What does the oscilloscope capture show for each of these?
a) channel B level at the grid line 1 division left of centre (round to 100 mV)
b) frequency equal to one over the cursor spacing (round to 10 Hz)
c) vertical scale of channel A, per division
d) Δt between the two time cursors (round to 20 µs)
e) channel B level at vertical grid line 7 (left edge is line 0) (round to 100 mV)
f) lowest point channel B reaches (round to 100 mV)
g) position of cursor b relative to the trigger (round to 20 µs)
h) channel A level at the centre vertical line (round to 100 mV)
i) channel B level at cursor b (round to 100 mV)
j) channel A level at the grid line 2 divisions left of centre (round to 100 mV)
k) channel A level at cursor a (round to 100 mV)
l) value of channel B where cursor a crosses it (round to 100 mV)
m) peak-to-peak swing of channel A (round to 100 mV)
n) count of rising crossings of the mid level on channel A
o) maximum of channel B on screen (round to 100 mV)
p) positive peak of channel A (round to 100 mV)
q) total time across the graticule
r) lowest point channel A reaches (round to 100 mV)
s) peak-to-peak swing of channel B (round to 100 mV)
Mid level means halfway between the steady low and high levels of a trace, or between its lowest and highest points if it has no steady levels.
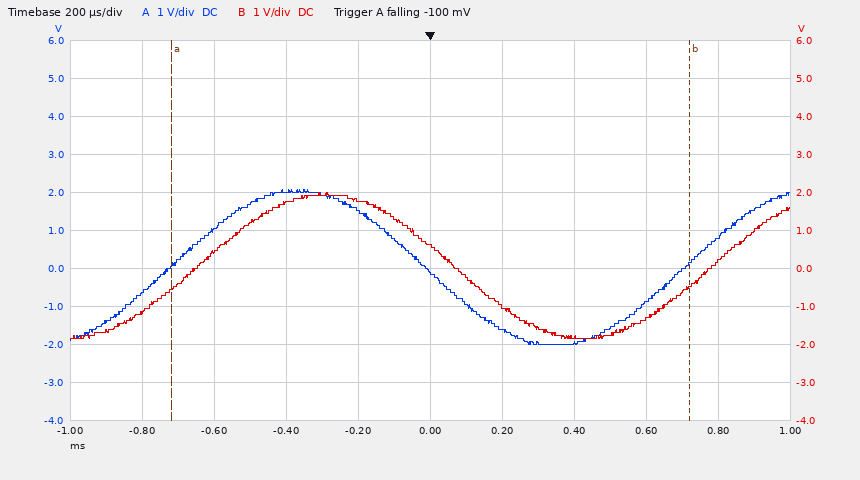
1.8 V
690 Hz
1 V
1.44 ms
-1.8 V
-1.8 V
+720 µs
-100 mV
-500 mV
2.0 V
100 mV
-600 mV
4.1 V
2
2.0 V
2.1 V
2 ms
-2.0 V
3.8 V
